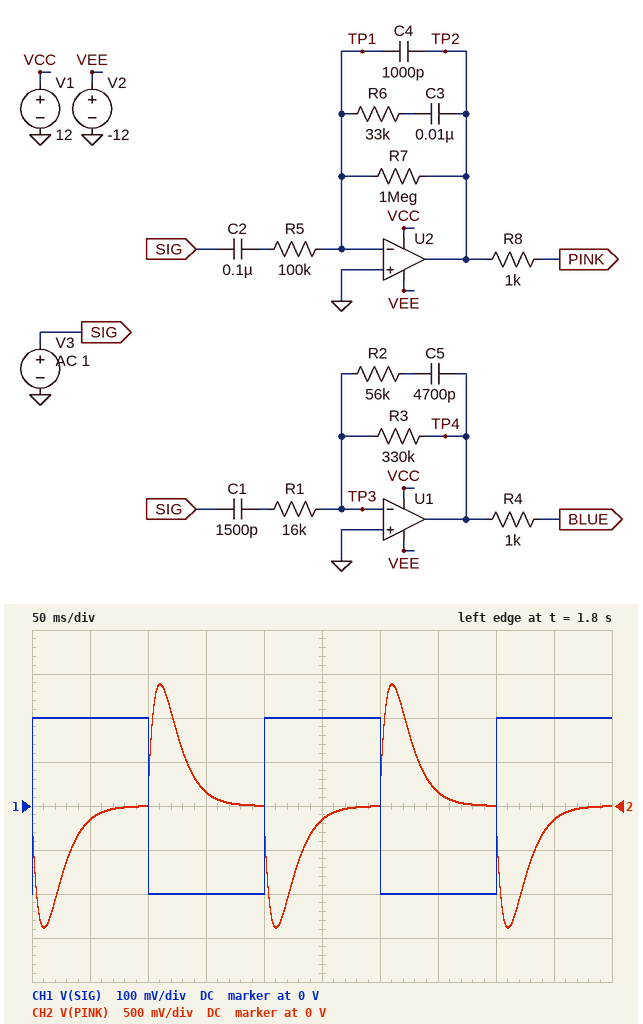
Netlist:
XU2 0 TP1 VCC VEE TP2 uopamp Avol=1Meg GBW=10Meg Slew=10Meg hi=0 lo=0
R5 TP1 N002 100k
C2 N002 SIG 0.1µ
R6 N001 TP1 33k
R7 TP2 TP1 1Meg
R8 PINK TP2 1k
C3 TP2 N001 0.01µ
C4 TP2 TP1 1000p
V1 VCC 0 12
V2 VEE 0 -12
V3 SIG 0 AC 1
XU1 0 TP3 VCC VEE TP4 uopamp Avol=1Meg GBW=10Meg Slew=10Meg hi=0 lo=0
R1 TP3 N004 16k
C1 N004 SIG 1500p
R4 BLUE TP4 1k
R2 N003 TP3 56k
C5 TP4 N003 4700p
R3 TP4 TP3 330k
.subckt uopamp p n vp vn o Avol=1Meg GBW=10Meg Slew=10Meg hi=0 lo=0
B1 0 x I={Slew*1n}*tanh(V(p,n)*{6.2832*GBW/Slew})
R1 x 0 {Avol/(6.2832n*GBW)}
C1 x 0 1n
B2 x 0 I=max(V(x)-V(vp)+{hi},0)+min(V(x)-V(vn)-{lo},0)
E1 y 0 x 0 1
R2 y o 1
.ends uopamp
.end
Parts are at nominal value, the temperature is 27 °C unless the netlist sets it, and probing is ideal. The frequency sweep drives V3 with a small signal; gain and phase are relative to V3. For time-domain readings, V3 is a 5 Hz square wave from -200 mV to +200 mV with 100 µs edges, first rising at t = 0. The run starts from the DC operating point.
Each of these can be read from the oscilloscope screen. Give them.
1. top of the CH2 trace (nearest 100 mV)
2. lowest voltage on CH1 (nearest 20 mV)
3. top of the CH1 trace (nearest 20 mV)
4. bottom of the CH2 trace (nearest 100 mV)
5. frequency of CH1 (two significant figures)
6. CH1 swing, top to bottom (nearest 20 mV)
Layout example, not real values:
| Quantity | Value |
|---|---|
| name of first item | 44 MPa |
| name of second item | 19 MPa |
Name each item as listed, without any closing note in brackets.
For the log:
| Quantity | Value |
|---|---|
| top of the CH2 trace | 1.4 V |
| lowest voltage on CH1 | -200 mV |
| top of the CH1 trace | 200 mV |
| bottom of the CH2 trace | -1.4 V |
| frequency of CH1 | 5.0 Hz |
| CH1 swing, top to bottom | 400 mV |
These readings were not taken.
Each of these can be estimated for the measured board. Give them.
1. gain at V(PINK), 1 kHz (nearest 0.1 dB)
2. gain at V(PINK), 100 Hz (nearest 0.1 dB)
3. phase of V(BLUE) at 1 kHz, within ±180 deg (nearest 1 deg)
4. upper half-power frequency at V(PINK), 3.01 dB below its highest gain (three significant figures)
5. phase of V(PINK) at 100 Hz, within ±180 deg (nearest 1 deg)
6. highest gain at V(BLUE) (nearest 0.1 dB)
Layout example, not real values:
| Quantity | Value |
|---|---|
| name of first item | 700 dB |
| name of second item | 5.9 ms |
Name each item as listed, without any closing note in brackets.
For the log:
| Quantity | Value |
|---|---|
| gain at V(PINK), 1 kHz | -9.9 dB |
| gain at V(PINK), 100 Hz | 3.0 dB |
| phase of V(BLUE) at 1 kHz, within ±180 deg | -125 deg |
| upper half-power frequency at V(PINK), 3.01 dB below its highest gain | 36.3 Hz |
| phase of V(PINK) at 100 Hz, within ±180 deg | 118 deg |
| highest gain at V(BLUE) | 9.5 dB |
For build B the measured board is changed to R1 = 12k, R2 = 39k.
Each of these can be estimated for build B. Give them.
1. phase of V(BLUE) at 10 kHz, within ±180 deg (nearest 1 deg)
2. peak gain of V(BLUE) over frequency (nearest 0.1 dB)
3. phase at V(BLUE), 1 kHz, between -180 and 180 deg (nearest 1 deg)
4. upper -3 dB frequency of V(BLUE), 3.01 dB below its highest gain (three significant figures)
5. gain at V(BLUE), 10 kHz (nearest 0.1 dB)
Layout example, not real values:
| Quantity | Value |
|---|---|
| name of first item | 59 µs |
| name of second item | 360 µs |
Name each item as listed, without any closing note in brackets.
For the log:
| Quantity | Value |
|---|---|
| phase of V(BLUE) at 10 kHz, within ±180 deg | -143 deg |
| peak gain of V(BLUE) over frequency | 9.3 dB |
| phase at V(BLUE), 1 kHz, between -180 and 180 deg | -132 deg |
| upper -3 dB frequency of V(BLUE), 3.01 dB below its highest gain | 2.57 MHz |
| gain at V(BLUE), 10 kHz | 6.8 dB |
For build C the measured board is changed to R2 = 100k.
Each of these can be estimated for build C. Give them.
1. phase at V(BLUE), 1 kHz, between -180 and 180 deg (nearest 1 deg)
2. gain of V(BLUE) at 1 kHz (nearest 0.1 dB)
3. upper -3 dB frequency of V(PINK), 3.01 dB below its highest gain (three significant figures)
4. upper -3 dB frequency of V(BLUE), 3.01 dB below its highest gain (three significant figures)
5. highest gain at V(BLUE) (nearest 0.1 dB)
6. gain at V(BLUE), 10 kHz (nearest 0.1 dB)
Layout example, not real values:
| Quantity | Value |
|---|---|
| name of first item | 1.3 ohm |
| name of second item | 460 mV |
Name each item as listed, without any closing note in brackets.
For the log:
| Quantity | Value |
|---|---|
| phase at V(BLUE), 1 kHz, between -180 and 180 deg | -113 deg |
| gain of V(BLUE) at 1 kHz | -2.5 dB |
| upper -3 dB frequency of V(PINK), 3.01 dB below its highest gain | 36.3 Hz |
| upper -3 dB frequency of V(BLUE), 3.01 dB below its highest gain | 1.73 MHz |
| highest gain at V(BLUE) | 13.6 dB |
| gain at V(BLUE), 10 kHz | 12.1 dB |
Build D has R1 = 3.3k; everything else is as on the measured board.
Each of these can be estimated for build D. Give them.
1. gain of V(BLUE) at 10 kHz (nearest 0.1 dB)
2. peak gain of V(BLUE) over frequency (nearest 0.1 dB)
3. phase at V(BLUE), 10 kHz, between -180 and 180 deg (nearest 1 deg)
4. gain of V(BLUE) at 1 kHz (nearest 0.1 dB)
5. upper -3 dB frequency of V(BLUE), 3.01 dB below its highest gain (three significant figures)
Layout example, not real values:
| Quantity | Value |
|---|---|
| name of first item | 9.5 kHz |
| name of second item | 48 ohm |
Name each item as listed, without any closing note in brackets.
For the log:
| Quantity | Value |
|---|---|
| gain of V(BLUE) at 10 kHz | 12.7 dB |
| peak gain of V(BLUE) over frequency | 23.2 dB |
| phase at V(BLUE), 10 kHz, between -180 and 180 deg | -110 deg |
| gain of V(BLUE) at 1 kHz | -5.6 dB |
| upper -3 dB frequency of V(BLUE), 3.01 dB below its highest gain | 678 kHz |
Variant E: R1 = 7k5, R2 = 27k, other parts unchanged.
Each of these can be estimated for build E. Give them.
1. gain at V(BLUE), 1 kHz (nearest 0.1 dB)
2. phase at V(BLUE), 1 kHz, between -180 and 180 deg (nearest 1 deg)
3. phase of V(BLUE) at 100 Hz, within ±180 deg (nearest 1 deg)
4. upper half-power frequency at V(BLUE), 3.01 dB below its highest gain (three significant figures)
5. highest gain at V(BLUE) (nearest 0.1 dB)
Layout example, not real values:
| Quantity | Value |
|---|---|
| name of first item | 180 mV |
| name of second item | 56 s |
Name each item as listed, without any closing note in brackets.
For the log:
| Quantity | Value |
|---|---|
| gain at V(BLUE), 1 kHz | -8.5 dB |
| phase at V(BLUE), 1 kHz, between -180 and 180 deg | -140 deg |
| phase of V(BLUE) at 100 Hz, within ±180 deg | -132 deg |
| upper half-power frequency at V(BLUE), 3.01 dB below its highest gain | 2.33 MHz |
| highest gain at V(BLUE) | 10.4 dB |
